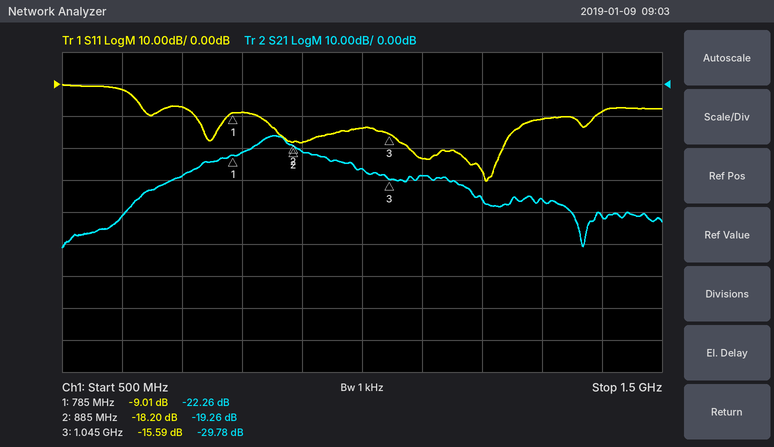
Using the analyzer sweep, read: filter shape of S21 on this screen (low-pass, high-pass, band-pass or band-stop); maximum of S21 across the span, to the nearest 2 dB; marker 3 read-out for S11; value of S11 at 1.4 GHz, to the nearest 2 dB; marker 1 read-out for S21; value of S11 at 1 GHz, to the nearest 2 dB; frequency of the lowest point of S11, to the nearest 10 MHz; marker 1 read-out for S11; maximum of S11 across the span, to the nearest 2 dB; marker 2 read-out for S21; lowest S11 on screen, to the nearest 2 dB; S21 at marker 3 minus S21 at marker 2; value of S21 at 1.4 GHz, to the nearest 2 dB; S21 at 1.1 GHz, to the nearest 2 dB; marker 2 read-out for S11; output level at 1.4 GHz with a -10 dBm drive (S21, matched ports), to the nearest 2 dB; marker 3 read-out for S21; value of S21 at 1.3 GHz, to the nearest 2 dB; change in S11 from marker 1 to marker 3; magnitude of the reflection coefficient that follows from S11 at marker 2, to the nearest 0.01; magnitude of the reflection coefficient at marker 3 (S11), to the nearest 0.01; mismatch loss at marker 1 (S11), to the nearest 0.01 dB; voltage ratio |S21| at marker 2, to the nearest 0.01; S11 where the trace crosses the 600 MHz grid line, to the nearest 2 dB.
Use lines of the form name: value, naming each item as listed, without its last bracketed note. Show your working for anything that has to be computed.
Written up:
filter shape of S21 on this screen: band-pass
maximum of S21 across the span, to the nearest 2 dB: -16 dB
marker 3 read-out for S11: -15.59 dB
value of S11 at 1.4 GHz, to the nearest 2 dB: -8 dB
marker 1 read-out for S21: -22.26 dB
value of S11 at 1 GHz, to the nearest 2 dB: -14 dB
frequency of the lowest point of S11, to the nearest 10 MHz: 1.21 GHz
marker 1 read-out for S11: -9.01 dB
maximum of S11 across the span, to the nearest 2 dB: 0 dB
marker 2 read-out for S21: -19.26 dB
lowest S11 on screen, to the nearest 2 dB: -30 dB
S21 at marker 3 minus S21 at marker 2: -29.78 − (-19.26) = -10.52 dB
value of S21 at 1.4 GHz, to the nearest 2 dB: -42 dB
S21 at 1.1 GHz, to the nearest 2 dB: -28 dB
marker 2 read-out for S11: -18.20 dB
output level at 1.4 GHz with a -10 dBm drive (S21, matched ports), to the nearest 2 dB: -10 dBm + (-42 dB) = -52 dBm
marker 3 read-out for S21: -29.78 dB
value of S21 at 1.3 GHz, to the nearest 2 dB: -36 dB
change in S11 from marker 1 to marker 3: -15.59 − (-9.01) = -6.58 dB
magnitude of the reflection coefficient that follows from S11 at marker 2, to the nearest 0.01: 10^(-18.2/20) ≈ 0.12
magnitude of the reflection coefficient at marker 3 (S11), to the nearest 0.01: 10^(-15.59/20) ≈ 0.17
mismatch loss at marker 1 (S11), to the nearest 0.01 dB: −10 log10(1 − 10^(-9.01/10)) ≈ 0.58 dB
voltage ratio |S21| at marker 2, to the nearest 0.01: 10^(-19.26/20) ≈ 0.11
S11 where the trace crosses the 600 MHz grid line, to the nearest 2 dB: -2 dB
